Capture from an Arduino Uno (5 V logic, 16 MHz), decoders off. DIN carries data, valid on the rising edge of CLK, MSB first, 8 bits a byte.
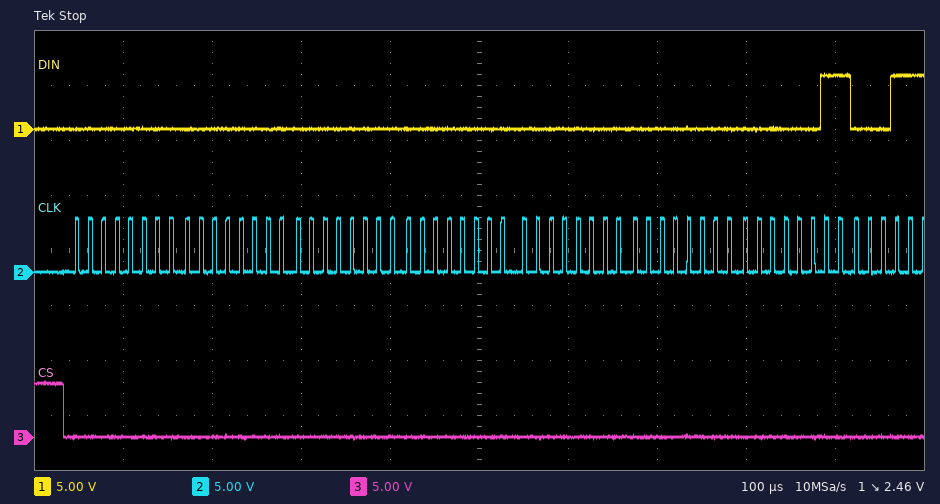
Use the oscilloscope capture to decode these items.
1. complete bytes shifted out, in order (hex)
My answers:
00 00 00 00 00 00 03
